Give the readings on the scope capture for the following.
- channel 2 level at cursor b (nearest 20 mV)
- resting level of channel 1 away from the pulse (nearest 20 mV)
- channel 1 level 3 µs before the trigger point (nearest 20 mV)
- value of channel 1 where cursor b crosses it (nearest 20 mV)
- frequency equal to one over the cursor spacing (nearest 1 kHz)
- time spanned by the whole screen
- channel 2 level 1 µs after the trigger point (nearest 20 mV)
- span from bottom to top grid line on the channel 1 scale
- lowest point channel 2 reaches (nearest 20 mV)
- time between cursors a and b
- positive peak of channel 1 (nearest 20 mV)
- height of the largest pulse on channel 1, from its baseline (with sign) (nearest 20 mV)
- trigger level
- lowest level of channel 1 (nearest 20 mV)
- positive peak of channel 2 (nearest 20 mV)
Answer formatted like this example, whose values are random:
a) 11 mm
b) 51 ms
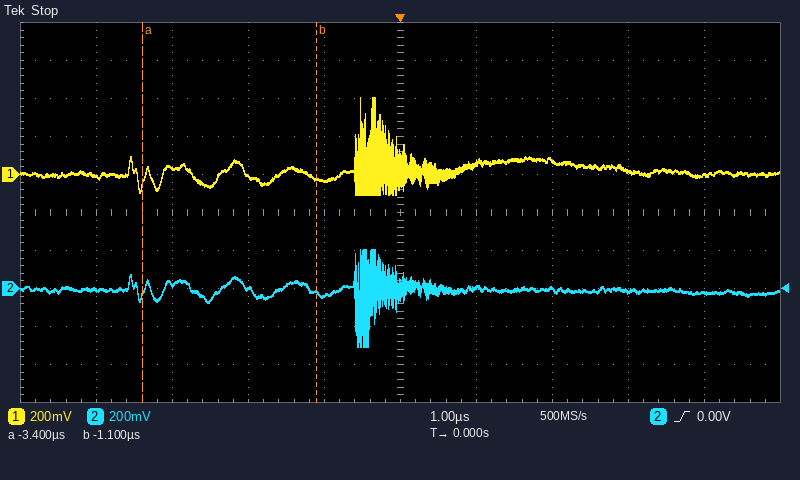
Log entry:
a) -20 mV
b) 0 mV
c) 40 mV
d) -20 mV
e) 435 kHz
f) 10 µs
g) 0 mV
h) 2 V
i) -300 mV
j) 2.3 µs
k) 400 mV
l) +400 mV
m) 0.00 V
n) -100 mV
o) 200 mV
